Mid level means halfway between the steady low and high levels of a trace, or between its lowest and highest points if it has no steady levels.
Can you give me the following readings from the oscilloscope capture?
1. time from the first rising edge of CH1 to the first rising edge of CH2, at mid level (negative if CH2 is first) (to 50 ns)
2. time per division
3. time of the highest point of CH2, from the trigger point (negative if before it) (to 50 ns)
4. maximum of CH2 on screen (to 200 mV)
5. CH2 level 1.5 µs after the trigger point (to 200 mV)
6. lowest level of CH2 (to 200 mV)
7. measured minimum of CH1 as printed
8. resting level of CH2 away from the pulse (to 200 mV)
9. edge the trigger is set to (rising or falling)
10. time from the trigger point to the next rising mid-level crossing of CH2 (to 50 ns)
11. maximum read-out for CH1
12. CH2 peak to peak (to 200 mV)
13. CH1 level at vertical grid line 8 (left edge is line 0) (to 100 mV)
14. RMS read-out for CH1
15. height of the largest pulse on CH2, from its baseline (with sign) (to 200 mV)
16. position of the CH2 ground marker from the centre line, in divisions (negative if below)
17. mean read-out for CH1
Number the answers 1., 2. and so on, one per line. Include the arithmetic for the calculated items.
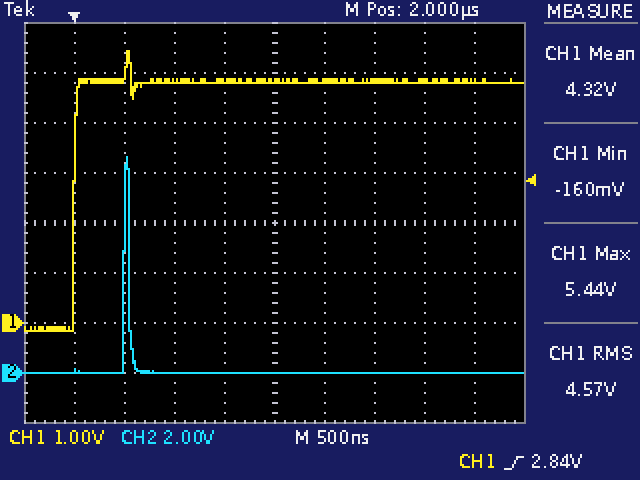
1. +500 ns
2. 500 ns
3. +550 ns
4. 8.6 V
5. 0.0 V
6. 0.0 V
7. -160 mV
8. 0.0 V
9. rising
10. 500 ns
11. 5.44 V
12. 8.6 V − (0.0 V) = 8.6 V
13. 4.8 V
14. 4.57 V
15. 8.6 V − (0.0 V) = +8.6 V
16. -3.0 div
17. 4.32 V
